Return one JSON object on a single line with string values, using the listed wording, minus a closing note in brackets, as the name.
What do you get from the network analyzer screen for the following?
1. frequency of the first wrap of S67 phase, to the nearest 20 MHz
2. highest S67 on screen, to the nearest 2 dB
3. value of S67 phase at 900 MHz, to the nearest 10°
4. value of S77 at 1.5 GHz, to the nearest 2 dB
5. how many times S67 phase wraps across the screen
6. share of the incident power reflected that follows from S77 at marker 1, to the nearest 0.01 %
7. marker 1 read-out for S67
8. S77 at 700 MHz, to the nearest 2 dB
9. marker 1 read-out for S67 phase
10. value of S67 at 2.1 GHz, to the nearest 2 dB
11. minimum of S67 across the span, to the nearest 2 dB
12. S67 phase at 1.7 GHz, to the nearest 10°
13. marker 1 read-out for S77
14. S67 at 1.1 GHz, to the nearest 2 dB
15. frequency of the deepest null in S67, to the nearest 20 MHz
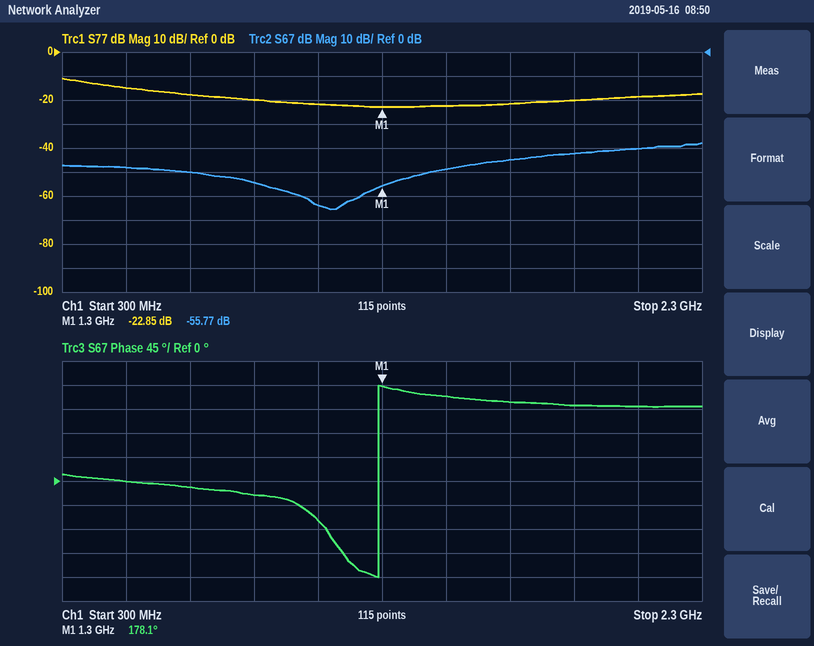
{"frequency of the first wrap of S67 phase, to the nearest 20 MHz": "1.28 GHz", "highest S67 on screen, to the nearest 2 dB": "-38 dB", "value of S67 phase at 900 MHz, to the nearest 10°": "-30°", "value of S77 at 1.5 GHz, to the nearest 2 dB": "-22 dB", "how many times S67 phase wraps across the screen": "1", "share of the incident power reflected that follows from S77 at marker 1, to the nearest 0.01 %": "0.52 %", "marker 1 read-out for S67": "-55.77 dB", "S77 at 700 MHz, to the nearest 2 dB": "-18 dB", "marker 1 read-out for S67 phase": "178.1°", "value of S67 at 2.1 GHz, to the nearest 2 dB": "-40 dB", "minimum of S67 across the span, to the nearest 2 dB": "-66 dB", "S67 phase at 1.7 GHz, to the nearest 10°": "150°", "marker 1 read-out for S77": "-22.85 dB", "S67 at 1.1 GHz, to the nearest 2 dB": "-64 dB", "frequency of the deepest null in S67, to the nearest 20 MHz": "1.14 GHz"}
